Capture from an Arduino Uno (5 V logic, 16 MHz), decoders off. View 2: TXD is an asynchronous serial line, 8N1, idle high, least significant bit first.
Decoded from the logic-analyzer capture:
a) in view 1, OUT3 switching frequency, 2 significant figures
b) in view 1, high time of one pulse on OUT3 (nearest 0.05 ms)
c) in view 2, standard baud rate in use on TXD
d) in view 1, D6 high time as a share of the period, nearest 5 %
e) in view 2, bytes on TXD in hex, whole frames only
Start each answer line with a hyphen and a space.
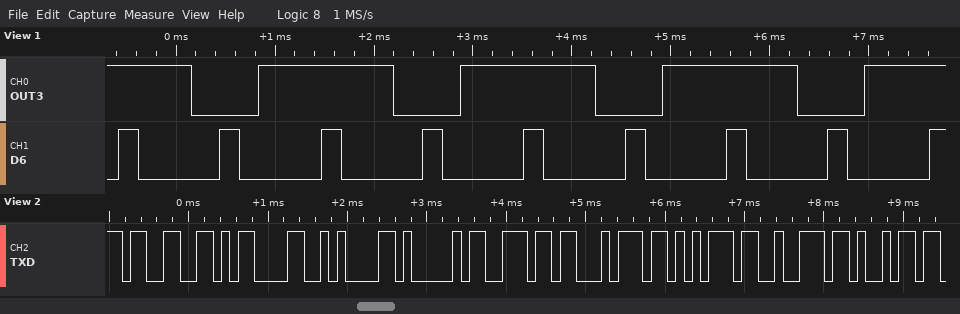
- 490 Hz
- 1.35 ms
- 9600 baud
- 20 %
- 33 0D 0A 41 6E 74 75 72 69
